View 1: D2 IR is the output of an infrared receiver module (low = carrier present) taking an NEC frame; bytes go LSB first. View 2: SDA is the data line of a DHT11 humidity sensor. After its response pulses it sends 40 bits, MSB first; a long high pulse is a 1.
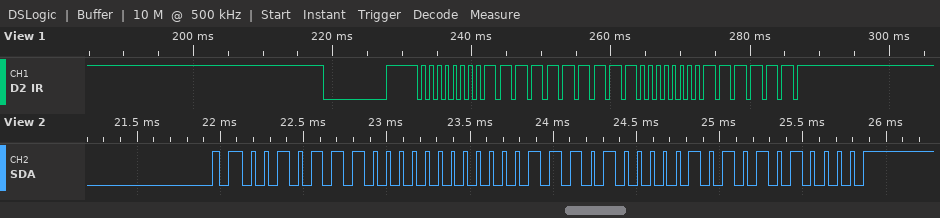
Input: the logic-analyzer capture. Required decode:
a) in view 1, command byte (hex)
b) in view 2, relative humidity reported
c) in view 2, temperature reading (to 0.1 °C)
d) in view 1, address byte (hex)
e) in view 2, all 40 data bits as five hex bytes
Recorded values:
0x03
46 %
29.5 °C
0x00
2E 00 1D 05 50
